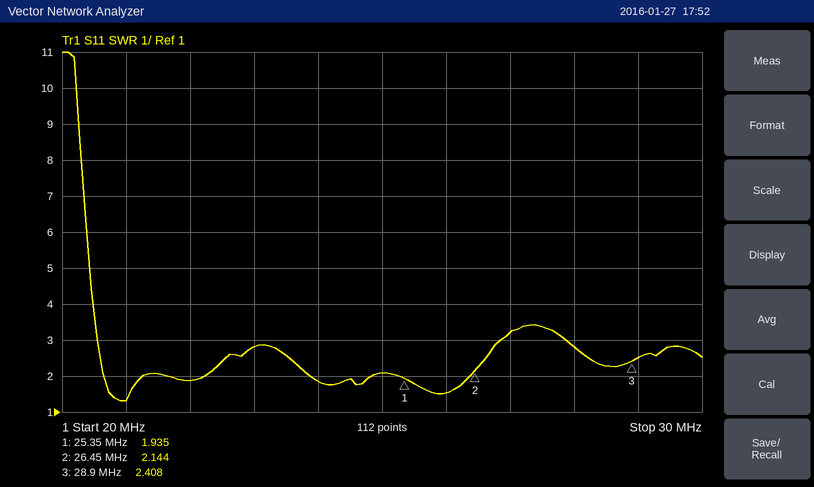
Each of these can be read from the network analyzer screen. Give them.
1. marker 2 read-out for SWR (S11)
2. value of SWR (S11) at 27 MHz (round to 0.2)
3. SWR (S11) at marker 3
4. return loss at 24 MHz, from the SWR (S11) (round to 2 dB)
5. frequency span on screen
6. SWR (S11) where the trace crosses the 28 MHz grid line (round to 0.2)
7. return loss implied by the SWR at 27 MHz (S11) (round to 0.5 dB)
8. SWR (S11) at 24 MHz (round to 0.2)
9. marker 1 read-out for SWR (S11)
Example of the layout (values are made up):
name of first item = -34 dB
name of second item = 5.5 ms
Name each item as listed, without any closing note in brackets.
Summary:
marker 2 read-out for SWR = 2.144
value of SWR (S11) at 27 MHz = 3.2
SWR (S11) at marker 3 = 2.408
return loss at 24 MHz, from the SWR (S11) = 10 dB
frequency span on screen = 10 MHz
SWR (S11) where the trace crosses the 28 MHz grid line = 2.8
return loss implied by the SWR at 27 MHz (S11) = 5.5 dB
SWR (S11) at 24 MHz = 1.8
marker 1 read-out for SWR = 1.935
